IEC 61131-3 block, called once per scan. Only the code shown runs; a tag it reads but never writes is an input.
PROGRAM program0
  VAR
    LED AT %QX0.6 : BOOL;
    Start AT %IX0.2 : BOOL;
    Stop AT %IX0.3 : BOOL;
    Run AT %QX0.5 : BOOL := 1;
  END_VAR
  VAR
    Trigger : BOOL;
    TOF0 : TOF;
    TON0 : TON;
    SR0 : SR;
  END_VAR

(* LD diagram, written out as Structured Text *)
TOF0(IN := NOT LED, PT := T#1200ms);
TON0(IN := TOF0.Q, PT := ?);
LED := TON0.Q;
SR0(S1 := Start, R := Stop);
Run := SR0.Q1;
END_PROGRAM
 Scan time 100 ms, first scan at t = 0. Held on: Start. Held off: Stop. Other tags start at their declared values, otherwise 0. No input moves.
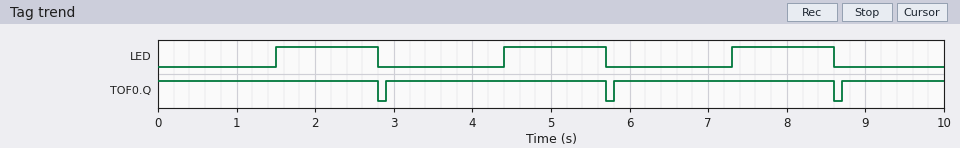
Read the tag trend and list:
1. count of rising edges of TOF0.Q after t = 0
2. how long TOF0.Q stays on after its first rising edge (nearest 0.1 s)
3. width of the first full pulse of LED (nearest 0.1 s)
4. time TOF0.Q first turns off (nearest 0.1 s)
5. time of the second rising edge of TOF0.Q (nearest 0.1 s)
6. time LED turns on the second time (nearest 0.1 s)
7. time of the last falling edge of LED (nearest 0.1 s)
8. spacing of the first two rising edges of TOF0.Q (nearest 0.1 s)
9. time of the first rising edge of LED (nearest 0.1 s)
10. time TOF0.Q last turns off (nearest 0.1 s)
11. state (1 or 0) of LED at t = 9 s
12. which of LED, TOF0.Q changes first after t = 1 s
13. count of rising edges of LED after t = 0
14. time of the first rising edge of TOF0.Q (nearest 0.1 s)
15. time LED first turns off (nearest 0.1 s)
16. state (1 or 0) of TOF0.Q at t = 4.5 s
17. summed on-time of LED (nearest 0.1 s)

3
2.8 s
1.3 s
2.8 s
5.8 s
4.4 s
8.6 s
2.9 s
1.5 s
8.6 s
0
LED
3
2.9 s
2.8 s
1
3.9 s
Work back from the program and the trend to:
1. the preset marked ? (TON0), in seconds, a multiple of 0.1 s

1.5 s
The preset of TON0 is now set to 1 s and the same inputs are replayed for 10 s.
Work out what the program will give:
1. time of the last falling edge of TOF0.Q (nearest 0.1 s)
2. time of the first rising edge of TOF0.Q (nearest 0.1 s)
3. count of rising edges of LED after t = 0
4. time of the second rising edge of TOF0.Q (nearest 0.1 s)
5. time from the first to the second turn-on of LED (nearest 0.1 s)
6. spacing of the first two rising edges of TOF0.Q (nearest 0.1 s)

9.5 s
2.4 s
4
4.8 s
2.4 s
2.4 s
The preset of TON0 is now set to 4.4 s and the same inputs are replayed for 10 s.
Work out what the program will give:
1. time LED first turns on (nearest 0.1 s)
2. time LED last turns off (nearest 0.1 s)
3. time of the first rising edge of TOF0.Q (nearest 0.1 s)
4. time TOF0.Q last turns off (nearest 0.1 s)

4.4 s
5.7 s
5.8 s
5.7 s
